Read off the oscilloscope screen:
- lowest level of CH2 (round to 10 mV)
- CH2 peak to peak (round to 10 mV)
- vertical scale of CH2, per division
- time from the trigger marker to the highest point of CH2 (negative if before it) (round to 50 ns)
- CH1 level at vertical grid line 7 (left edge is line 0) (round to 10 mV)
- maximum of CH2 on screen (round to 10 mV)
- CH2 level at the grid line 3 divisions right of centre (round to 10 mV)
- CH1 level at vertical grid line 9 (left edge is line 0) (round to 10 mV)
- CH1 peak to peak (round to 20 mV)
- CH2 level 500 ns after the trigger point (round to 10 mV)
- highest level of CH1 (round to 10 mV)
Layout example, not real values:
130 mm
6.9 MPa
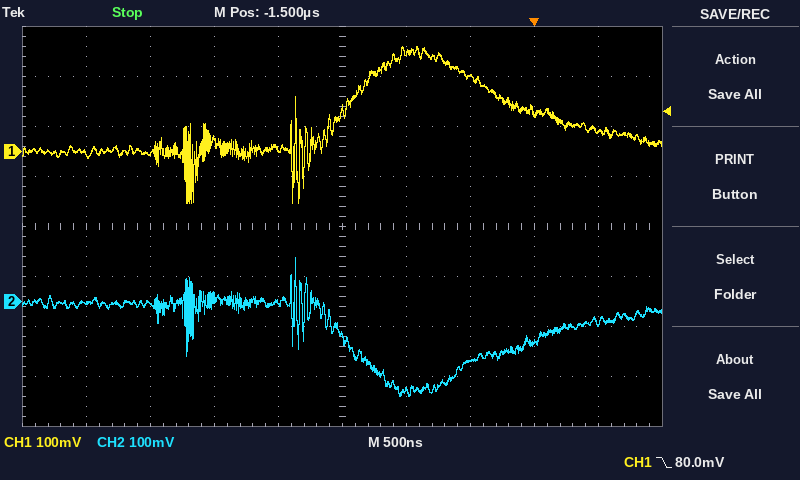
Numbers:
-190 mV
280 mV
100 mV
-1.85 µs
150 mV
90 mV
-80 mV
40 mV
320 mV
-40 mV
210 mV
